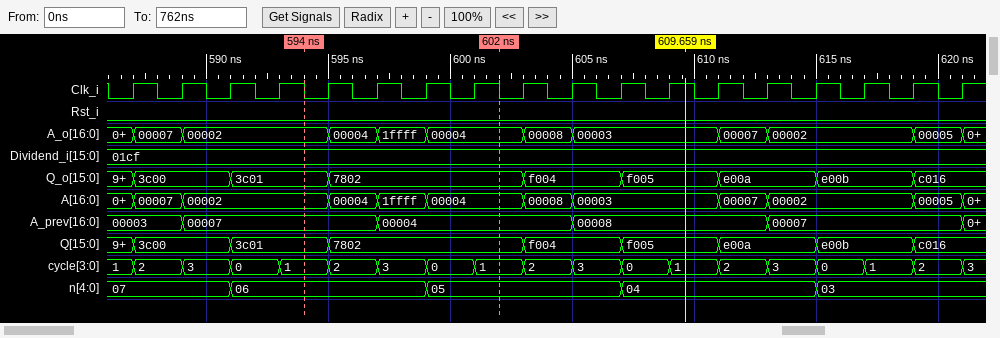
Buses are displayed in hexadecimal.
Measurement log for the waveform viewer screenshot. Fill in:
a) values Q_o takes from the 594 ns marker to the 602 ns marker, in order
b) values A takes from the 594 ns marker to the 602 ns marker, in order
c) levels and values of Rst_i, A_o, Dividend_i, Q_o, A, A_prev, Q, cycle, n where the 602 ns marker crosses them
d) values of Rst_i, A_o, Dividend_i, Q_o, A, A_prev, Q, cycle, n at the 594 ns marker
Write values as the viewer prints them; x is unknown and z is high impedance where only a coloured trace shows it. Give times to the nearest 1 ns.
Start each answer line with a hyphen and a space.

- 3c01, 7802
- 00002, 00004, 1ffff, 00004
- Rst_i=0, A_o=00004, Dividend_i=01cf, Q_o=7802, A=00004, A_prev=00004, Q=7802, cycle=1, n=05
- Rst_i=0, A_o=00002, Dividend_i=01cf, Q_o=3c01, A=00002, A_prev=00007, Q=3c01, cycle=1, n=06
